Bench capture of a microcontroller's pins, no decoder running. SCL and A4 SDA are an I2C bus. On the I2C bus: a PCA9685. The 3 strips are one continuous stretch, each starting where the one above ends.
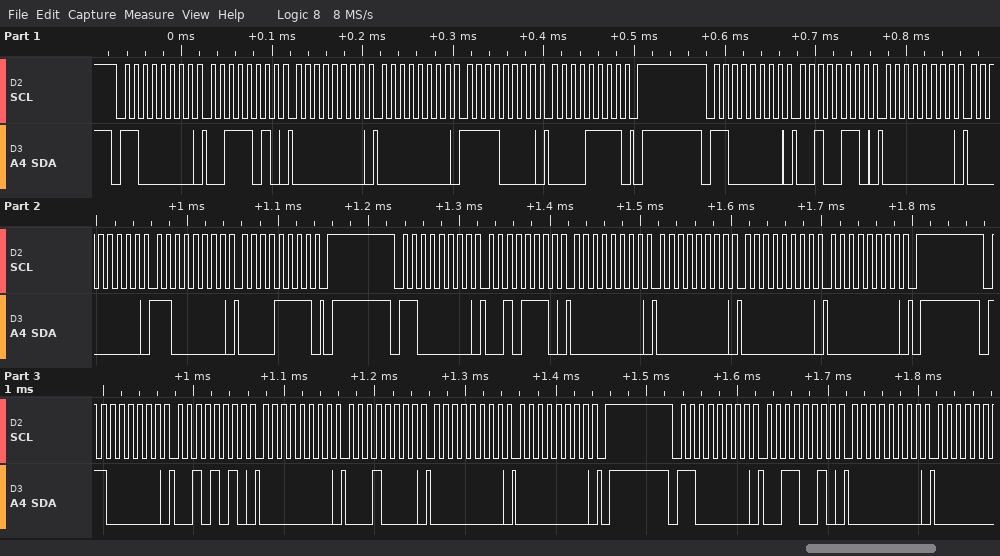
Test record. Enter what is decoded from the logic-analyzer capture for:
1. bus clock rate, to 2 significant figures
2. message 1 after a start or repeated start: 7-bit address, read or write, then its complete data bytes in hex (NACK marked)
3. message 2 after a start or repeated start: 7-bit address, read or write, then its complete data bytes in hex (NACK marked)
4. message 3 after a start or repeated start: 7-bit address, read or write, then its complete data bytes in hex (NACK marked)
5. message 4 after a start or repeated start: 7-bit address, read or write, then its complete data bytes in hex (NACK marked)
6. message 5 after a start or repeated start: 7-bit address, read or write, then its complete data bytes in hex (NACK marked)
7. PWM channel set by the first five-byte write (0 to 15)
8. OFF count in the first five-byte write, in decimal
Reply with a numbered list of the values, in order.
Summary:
1. 100 kHz
2. 0x60 write: 3A 00 00 F0 0F
3. 0x60 write: 26 00 00 C0 0F
4. 0x60 write: 2E 00 00 00 00
5. 0x60 write: 2A 00 10 00 00
6. 0x60 write: 32 00
7. 13
8. 4080
